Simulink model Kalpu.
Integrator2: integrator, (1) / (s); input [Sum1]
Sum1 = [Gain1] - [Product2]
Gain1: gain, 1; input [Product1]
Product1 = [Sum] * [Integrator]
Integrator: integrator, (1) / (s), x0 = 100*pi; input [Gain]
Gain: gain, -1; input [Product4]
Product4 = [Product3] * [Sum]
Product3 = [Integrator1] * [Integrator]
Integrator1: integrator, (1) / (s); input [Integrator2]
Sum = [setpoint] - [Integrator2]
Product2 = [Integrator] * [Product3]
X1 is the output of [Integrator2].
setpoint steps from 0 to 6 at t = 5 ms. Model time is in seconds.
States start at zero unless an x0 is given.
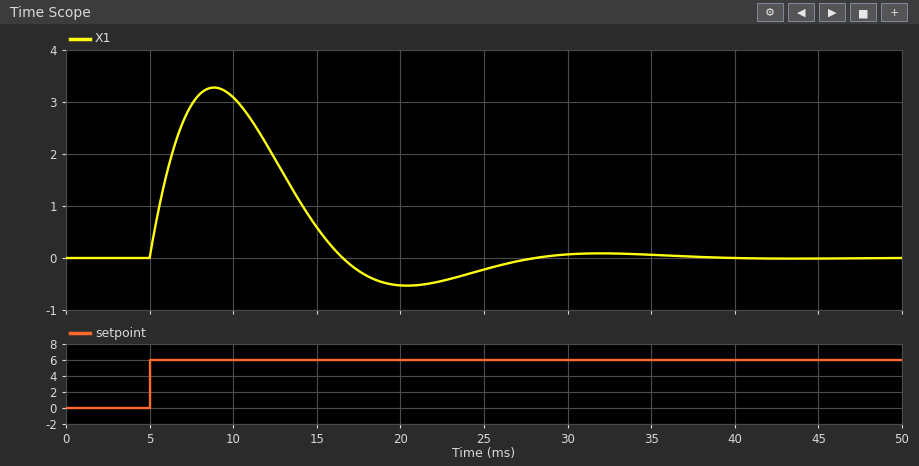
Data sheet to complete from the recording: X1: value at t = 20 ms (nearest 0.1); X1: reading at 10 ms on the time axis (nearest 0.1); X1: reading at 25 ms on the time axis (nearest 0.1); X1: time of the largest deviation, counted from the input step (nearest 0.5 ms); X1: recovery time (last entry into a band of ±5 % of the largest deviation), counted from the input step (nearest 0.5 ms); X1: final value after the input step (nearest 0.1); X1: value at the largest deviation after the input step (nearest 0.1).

-0.5
3.1
-0.2
4.0 ms
20.5 ms
0.0
3.3
